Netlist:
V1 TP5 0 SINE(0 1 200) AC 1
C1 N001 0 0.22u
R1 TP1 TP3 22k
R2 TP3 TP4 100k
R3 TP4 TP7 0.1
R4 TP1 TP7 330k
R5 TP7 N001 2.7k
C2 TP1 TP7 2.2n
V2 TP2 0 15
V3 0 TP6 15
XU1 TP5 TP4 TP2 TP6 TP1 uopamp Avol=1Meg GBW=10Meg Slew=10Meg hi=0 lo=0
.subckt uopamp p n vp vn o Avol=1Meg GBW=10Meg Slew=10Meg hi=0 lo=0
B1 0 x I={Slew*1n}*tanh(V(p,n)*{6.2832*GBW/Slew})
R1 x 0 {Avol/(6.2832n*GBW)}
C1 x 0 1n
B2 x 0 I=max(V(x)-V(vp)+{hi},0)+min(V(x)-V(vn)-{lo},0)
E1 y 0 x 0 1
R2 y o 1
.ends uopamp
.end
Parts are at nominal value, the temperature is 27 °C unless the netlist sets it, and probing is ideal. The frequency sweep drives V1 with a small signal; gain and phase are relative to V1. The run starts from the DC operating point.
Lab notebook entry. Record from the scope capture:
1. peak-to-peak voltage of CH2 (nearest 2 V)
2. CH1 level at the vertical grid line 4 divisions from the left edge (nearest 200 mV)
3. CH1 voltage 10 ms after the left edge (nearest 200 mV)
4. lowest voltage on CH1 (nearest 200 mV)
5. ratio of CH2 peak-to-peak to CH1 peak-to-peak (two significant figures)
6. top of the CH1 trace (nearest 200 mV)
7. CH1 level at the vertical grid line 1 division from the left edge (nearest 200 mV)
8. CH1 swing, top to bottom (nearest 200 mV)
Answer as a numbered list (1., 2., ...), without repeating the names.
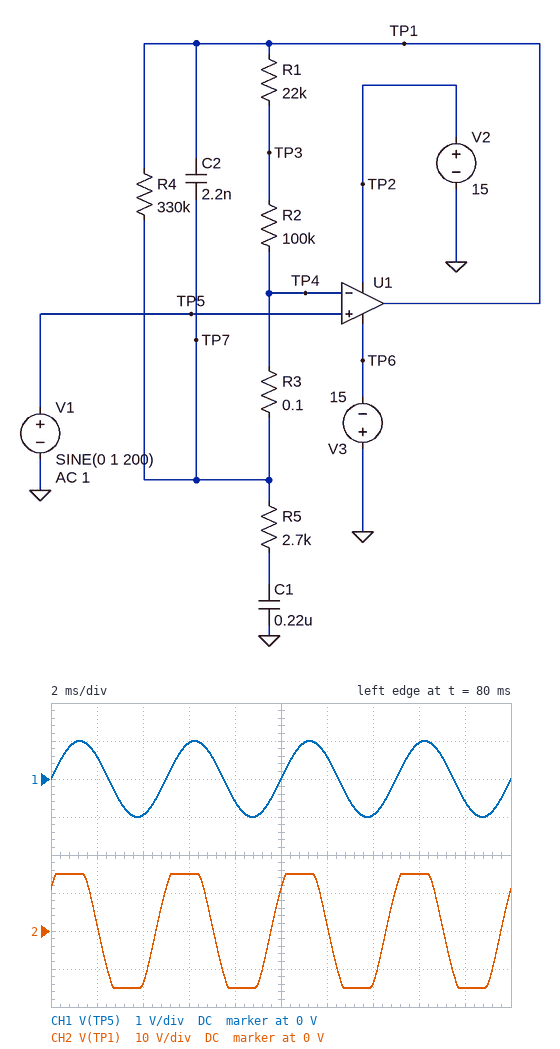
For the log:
1. 30 V
2. -600 mV
3. 0 V
4. -1.0 V
5. 15
6. 1.0 V
7. 600 mV
8. 2.0 V
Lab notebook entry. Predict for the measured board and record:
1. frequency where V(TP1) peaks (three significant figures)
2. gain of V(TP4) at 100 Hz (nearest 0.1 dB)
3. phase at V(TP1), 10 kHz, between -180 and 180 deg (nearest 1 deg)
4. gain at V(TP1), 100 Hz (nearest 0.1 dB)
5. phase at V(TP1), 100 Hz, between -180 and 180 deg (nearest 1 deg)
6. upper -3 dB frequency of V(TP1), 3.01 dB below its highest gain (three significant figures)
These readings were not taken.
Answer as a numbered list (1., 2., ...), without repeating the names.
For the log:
1. 466 Hz
2. 0 dB
3. -64 deg
4. 21.5 dB
5. 58 deg
6. 1.25 kHz
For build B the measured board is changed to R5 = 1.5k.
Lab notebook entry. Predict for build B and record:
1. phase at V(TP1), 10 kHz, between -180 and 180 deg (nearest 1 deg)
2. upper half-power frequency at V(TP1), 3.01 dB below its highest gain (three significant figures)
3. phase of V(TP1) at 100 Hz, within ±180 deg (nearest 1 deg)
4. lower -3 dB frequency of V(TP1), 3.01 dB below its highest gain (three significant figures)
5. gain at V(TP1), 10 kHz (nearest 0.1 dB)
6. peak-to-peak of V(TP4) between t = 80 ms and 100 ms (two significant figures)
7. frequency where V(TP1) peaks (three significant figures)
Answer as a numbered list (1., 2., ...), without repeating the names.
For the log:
1. -71 deg
2. 1.54 kHz
3. 67 deg
4. 253 Hz
5. 14.0 dB
6. 1.9 V
7. 624 Hz
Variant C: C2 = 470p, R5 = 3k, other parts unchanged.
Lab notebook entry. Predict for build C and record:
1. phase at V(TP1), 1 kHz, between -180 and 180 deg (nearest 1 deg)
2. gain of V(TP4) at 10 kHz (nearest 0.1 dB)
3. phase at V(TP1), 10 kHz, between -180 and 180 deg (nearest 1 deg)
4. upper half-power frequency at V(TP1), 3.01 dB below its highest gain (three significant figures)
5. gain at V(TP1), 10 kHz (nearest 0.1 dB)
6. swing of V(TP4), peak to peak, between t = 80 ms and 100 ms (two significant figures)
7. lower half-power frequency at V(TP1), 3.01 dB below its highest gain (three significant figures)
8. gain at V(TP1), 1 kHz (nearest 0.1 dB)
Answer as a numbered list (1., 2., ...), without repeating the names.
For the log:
1. -1 deg
2. -0.1 dB
3. -63 deg
4. 4.22 kHz
5. 20.7 dB
6. 2.0 V
7. 215 Hz
8. 29.2 dB
